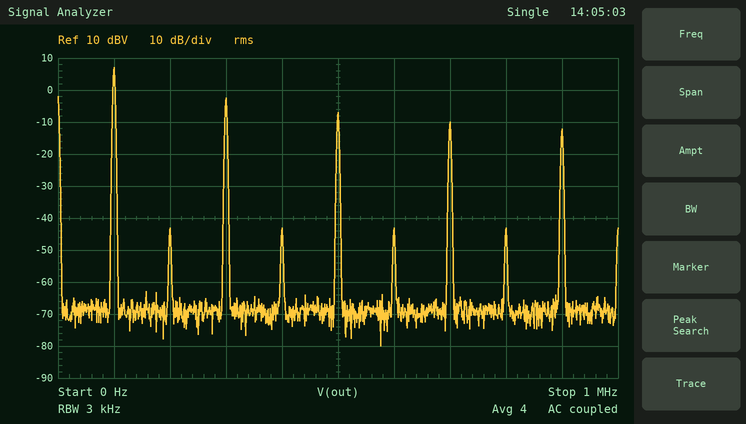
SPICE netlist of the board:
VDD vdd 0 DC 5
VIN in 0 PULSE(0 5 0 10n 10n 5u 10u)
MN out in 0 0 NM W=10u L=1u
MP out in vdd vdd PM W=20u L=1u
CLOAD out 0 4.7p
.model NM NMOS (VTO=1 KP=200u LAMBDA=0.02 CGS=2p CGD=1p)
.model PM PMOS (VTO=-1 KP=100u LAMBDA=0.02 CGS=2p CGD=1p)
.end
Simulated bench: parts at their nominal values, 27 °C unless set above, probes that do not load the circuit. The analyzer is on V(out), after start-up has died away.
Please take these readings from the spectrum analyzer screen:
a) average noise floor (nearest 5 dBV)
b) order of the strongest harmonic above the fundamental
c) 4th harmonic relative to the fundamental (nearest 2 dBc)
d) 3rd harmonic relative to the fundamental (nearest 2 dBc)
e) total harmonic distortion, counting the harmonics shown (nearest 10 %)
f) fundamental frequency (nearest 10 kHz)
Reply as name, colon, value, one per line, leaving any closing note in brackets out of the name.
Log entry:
average noise floor: -70 dBV
order of the strongest harmonic above the fundamental: 3
4th harmonic relative to the fundamental: -50 dBc
3rd harmonic relative to the fundamental: -10 dBc
total harmonic distortion, counting the harmonics shown: 40 %
fundamental frequency: 100 kHz
